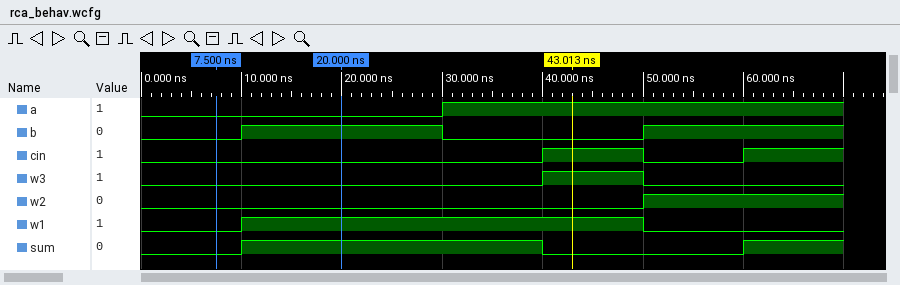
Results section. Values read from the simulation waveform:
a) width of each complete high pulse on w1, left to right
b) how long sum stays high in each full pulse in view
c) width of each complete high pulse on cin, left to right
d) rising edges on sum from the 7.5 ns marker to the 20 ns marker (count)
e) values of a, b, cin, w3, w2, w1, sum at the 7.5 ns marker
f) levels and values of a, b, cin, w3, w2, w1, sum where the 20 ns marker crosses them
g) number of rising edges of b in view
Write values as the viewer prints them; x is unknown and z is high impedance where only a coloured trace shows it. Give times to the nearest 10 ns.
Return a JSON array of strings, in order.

["40 ns", "30 ns", "10 ns", "1", "a=0, b=0, cin=0, w3=0, w2=0, w1=0, sum=0", "a=0, b=1, cin=0, w3=0, w2=0, w1=1, sum=1", "2"]
